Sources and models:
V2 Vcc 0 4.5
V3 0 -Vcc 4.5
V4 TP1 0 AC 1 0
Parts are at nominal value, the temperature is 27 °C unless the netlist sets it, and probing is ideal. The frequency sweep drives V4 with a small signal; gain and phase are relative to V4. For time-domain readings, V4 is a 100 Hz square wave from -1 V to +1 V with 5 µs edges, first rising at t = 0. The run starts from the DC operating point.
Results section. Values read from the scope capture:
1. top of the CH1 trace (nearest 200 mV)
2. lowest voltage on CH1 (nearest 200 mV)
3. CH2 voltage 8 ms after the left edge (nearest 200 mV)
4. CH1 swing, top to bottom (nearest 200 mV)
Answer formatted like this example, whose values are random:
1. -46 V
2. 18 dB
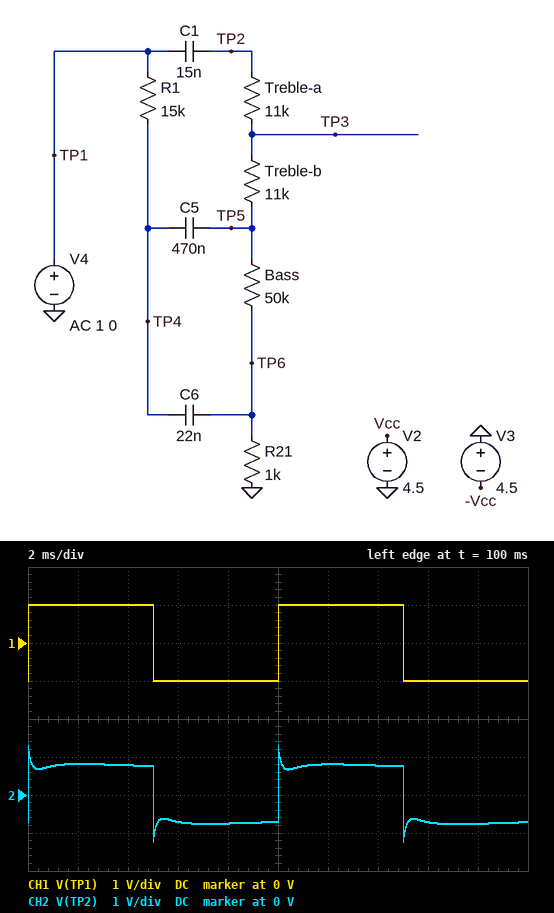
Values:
1. 1.0 V
2. -1.0 V
3. -800 mV
4. 2.0 V
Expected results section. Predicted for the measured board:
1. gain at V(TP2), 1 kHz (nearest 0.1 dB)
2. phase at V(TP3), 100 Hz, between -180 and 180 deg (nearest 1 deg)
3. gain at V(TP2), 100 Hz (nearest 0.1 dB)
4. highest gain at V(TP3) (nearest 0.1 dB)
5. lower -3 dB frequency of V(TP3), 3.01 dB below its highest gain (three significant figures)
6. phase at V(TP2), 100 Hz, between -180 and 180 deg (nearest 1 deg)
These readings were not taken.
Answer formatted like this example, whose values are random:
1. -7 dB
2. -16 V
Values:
1. -2.1 dB
2. -2 deg
3. -2.3 dB
4. -2.2 dB
5. 4.90 Hz
6. 0 deg
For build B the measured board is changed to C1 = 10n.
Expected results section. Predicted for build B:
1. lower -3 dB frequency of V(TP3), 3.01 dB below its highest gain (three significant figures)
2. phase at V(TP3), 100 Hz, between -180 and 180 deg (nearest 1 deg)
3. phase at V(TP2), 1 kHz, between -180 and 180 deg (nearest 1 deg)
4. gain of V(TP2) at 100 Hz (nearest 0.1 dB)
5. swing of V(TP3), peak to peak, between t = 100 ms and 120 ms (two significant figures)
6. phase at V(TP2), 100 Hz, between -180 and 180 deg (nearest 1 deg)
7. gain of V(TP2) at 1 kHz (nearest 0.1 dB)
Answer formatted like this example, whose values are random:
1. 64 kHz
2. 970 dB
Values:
1. 4.93 Hz
2. -3 deg
3. 16 deg
4. -2.4 dB
5. 1.6 V
6. -2 deg
7. -3.3 dB
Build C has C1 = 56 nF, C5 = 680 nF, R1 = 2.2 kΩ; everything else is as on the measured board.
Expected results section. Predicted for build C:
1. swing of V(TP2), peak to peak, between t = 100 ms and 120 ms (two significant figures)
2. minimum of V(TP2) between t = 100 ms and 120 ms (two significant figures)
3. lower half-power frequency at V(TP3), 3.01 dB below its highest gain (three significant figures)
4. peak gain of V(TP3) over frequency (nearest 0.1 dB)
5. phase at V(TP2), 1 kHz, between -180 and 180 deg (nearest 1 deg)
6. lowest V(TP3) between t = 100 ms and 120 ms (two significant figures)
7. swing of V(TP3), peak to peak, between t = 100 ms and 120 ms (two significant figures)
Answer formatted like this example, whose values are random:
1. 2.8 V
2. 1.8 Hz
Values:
1. 2.2 V
2. -1.0 V
3. 4.04 Hz
4. -0.2 dB
5. 1 deg
6. -960 mV
7. 2.0 V
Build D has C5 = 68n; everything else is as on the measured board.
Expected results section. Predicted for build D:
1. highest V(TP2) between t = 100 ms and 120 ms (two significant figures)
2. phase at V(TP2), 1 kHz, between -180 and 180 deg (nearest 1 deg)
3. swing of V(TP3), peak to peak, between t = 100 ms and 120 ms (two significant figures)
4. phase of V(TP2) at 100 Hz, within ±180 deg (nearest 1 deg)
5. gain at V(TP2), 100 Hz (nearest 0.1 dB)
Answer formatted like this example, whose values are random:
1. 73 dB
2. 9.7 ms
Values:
1. 1.5 V
2. 11 deg
3. 1.9 V
4. 13 deg
5. -1.8 dB
